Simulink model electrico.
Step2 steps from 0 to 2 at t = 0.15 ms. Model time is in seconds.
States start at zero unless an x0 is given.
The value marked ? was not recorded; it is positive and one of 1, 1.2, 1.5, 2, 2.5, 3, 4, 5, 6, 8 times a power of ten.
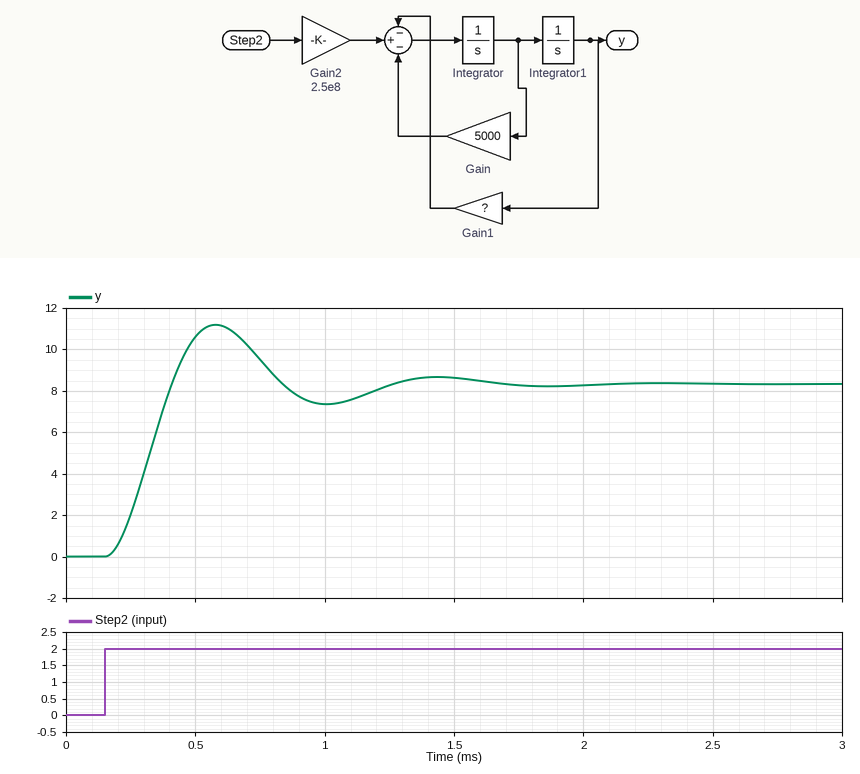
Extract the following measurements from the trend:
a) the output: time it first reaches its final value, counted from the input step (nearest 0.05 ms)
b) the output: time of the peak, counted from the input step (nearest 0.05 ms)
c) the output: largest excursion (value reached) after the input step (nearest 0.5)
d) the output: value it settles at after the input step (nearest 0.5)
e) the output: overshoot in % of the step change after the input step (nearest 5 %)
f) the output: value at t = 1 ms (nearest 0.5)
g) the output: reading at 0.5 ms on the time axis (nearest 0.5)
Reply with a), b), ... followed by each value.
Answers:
a) 0.25 ms
b) 0.45 ms
c) 11.0
d) 8.5
e) 35 %
f) 7.5
g) 10.5
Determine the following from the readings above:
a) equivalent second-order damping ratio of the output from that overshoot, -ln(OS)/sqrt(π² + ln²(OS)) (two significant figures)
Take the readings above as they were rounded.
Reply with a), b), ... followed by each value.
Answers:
a) 0.32
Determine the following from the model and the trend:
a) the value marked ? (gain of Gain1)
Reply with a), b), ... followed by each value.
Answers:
a) 6e+07
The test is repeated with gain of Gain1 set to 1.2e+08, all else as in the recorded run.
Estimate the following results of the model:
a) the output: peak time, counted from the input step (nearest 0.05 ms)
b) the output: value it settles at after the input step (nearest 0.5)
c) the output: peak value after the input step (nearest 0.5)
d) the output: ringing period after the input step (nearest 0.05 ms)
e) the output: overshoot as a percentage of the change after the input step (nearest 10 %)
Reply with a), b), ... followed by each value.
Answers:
a) 0.30 ms
b) 4.0
c) 6.0
d) 0.60 ms
e) 50 %
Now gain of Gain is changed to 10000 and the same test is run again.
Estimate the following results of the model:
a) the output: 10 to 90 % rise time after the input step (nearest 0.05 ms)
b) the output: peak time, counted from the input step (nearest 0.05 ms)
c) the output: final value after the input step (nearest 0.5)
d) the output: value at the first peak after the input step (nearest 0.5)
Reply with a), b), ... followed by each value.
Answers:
a) 0.25 ms
b) 0.55 ms
c) 8.5
d) 9.0
